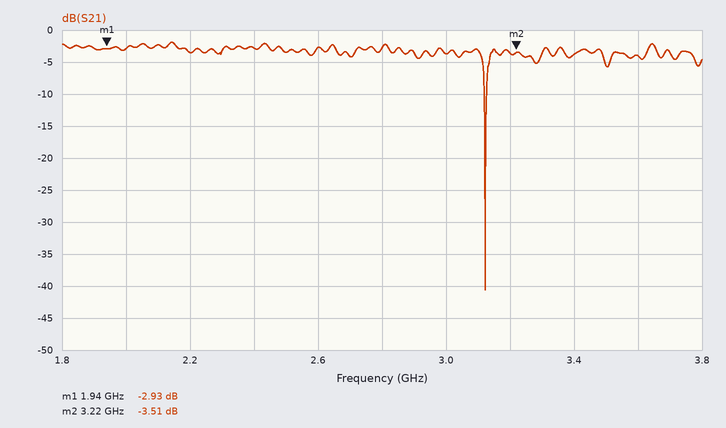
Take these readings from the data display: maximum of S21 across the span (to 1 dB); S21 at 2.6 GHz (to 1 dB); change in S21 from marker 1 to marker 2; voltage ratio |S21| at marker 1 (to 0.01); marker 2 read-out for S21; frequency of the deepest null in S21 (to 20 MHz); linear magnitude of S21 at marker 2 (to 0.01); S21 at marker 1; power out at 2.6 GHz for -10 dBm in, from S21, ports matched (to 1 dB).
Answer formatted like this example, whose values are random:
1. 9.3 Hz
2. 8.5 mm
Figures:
1. -2 dB
2. -3 dB
3. -0.58 dB
4. 0.71
5. -3.51 dB
6. 3.12 GHz
7. 0.67
8. -2.93 dB
9. -13 dBm
